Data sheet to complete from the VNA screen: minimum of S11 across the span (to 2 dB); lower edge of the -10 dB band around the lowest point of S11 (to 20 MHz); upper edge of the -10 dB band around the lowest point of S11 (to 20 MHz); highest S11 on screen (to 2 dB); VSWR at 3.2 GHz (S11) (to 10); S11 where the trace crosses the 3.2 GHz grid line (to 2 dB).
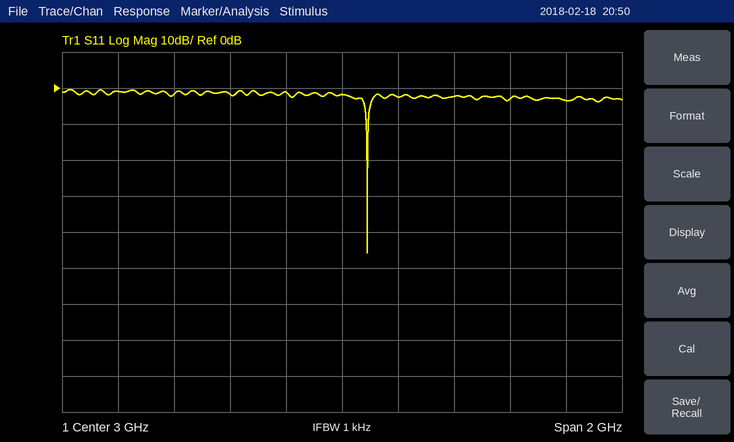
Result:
-46 dB
3.08 GHz
3.10 GHz
0 dB
10
-2 dB
